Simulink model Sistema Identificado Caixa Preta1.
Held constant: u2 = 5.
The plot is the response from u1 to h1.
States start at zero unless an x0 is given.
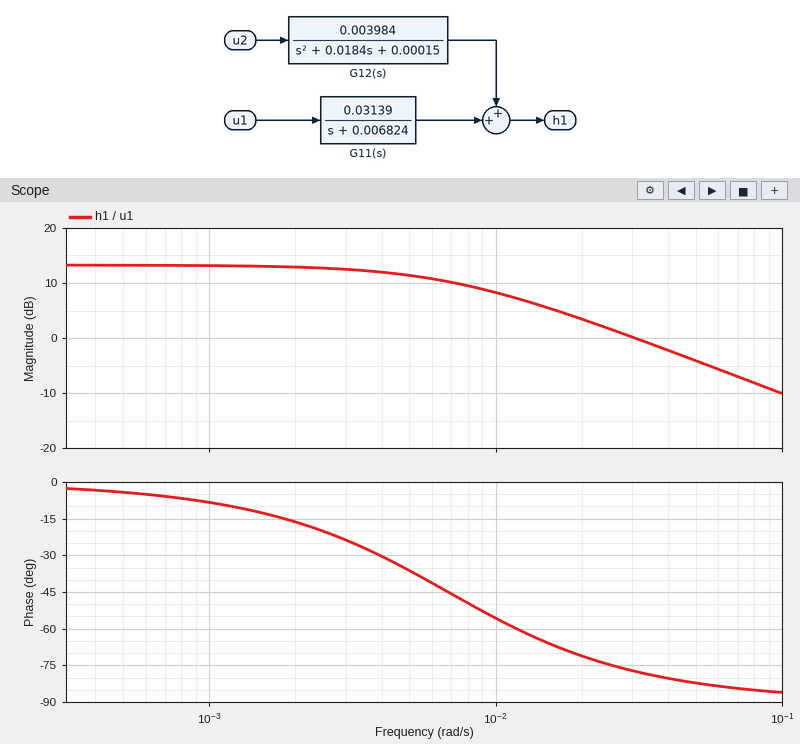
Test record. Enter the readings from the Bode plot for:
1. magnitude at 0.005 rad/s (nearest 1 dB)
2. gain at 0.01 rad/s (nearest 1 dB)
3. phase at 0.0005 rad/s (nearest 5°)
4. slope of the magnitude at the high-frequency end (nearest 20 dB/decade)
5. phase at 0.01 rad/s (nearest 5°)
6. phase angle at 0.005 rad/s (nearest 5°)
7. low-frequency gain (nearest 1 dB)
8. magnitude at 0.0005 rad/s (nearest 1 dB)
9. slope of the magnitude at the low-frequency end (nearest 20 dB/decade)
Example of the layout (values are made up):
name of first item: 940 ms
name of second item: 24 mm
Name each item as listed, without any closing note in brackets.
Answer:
magnitude at 0.005 rad/s: 11 dB
gain at 0.01 rad/s: 8 dB
phase at 0.0005 rad/s: -5°
slope of the magnitude at the high-frequency end: -20 dB/decade
phase at 0.01 rad/s: -55°
phase angle at 0.005 rad/s: -35°
low-frequency gain: 13 dB
magnitude at 0.0005 rad/s: 13 dB
slope of the magnitude at the low-frequency end: 0 dB/decade
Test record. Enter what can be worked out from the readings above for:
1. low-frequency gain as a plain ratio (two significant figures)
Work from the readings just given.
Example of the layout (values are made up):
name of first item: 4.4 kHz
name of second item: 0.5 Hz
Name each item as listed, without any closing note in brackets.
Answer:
low-frequency gain as a plain ratio: 4.5
